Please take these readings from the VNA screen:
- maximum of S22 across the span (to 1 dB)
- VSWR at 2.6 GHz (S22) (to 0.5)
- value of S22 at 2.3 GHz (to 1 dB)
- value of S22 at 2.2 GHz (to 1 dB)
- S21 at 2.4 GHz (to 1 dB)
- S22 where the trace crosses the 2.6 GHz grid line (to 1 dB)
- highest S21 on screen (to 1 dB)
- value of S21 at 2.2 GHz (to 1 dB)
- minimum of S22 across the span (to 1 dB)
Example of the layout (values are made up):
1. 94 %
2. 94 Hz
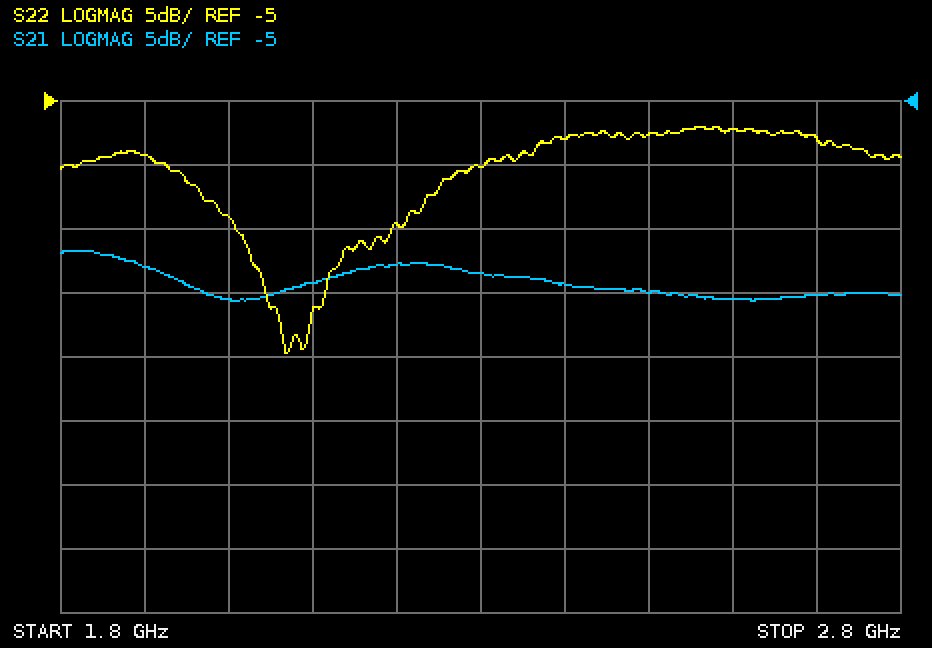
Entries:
1. -7 dB
2. 2.5
3. -10 dB
4. -15 dB
5. -19 dB
6. -7 dB
7. -17 dB
8. -18 dB
9. -25 dB
